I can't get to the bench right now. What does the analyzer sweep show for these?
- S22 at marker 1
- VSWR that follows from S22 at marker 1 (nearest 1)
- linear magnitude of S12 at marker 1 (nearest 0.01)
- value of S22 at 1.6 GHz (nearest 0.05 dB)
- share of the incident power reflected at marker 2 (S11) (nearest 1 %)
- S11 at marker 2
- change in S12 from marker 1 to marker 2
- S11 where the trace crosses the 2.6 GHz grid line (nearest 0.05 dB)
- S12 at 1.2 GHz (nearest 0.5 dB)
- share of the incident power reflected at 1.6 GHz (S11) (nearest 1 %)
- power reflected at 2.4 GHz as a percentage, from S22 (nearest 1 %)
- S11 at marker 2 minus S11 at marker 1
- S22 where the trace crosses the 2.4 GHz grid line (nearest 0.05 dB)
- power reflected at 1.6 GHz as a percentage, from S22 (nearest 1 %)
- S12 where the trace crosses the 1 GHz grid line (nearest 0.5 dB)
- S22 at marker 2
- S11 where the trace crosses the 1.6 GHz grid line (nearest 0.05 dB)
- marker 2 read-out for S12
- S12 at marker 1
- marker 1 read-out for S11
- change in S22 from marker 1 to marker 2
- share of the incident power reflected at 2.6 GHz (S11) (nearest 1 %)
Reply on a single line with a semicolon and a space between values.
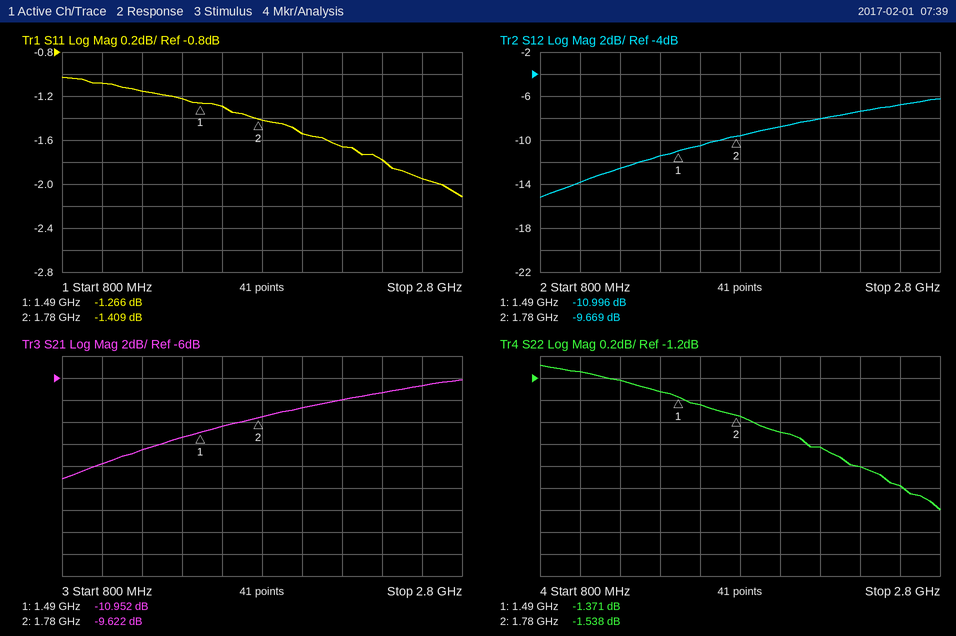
-1.371 dB; 13; 0.28; -1.45 dB; 72 %; -1.409 dB; 1.327 dB; -1.95 dB; -12.5 dB; 74 %; 63 %; -0.143 dB; -2.00 dB; 72 %; -14.0 dB; -1.538 dB; -1.30 dB; -9.669 dB; -10.996 dB; -1.266 dB; -0.167 dB; 64 %
